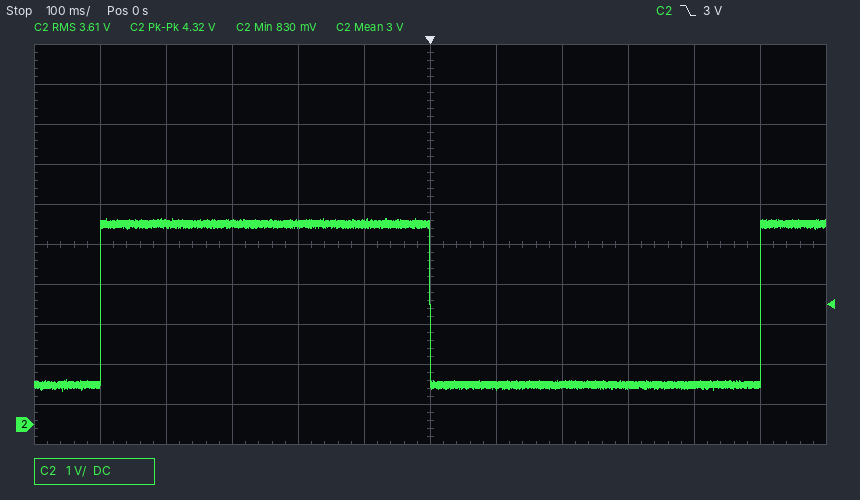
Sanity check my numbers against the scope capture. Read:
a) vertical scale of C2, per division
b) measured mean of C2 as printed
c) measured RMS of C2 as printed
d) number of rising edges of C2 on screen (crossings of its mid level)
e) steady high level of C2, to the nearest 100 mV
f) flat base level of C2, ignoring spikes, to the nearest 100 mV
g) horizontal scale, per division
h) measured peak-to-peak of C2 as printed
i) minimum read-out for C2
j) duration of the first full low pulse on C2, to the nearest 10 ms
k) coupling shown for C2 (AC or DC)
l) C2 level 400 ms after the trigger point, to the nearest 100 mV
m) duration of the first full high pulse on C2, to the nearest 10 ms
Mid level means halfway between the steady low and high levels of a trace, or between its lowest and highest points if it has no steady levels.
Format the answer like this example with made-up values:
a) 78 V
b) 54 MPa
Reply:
a) 1 V
b) 3 V
c) 3.61 V
d) 2
e) 5.0 V
f) 1.0 V
g) 100 ms
h) 4.32 V
i) 830 mV
j) 500 ms
k) DC
l) 1.0 V
m) 500 ms
